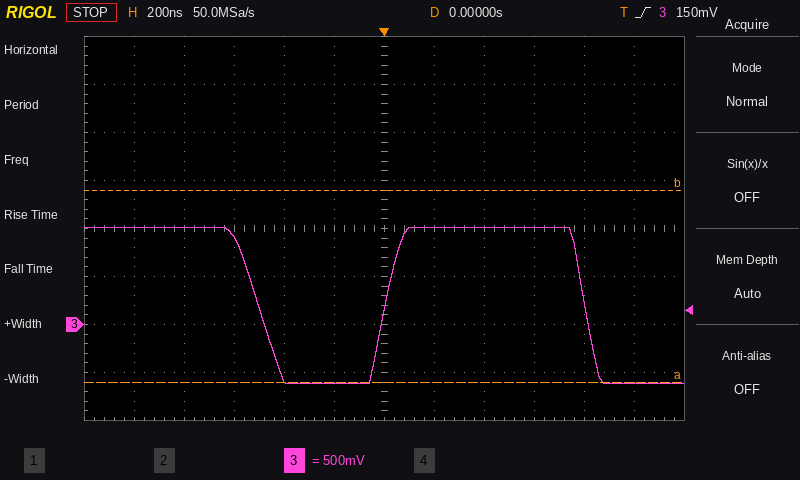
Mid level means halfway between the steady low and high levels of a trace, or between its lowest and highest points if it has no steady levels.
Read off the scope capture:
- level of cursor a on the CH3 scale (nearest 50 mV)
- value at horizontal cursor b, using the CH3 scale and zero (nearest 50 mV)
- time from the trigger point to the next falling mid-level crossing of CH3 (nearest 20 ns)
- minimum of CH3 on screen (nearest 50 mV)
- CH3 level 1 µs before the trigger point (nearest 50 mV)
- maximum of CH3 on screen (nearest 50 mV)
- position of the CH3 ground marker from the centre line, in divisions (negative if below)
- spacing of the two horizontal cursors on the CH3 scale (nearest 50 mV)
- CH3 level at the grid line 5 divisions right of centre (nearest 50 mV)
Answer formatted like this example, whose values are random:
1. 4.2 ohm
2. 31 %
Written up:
1. -600 mV
2. 1.40 V
3. 800 ns
4. -600 mV
5. 1.00 V
6. 1.00 V
7. -2.0 div
8. 2.00 V
9. -600 mV
